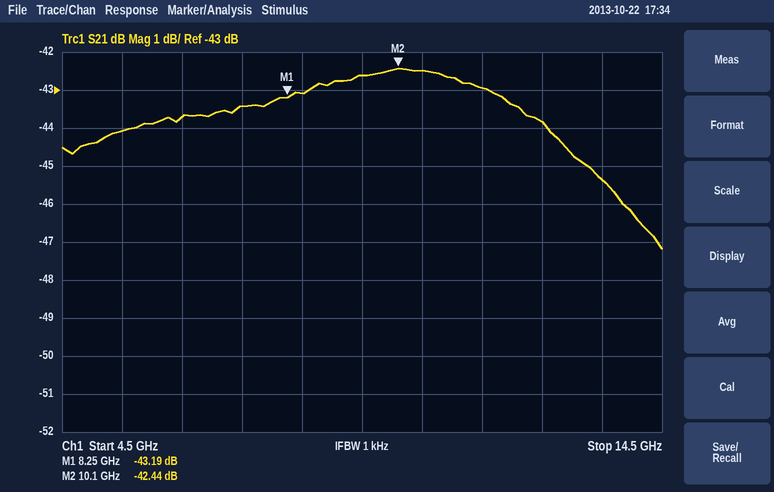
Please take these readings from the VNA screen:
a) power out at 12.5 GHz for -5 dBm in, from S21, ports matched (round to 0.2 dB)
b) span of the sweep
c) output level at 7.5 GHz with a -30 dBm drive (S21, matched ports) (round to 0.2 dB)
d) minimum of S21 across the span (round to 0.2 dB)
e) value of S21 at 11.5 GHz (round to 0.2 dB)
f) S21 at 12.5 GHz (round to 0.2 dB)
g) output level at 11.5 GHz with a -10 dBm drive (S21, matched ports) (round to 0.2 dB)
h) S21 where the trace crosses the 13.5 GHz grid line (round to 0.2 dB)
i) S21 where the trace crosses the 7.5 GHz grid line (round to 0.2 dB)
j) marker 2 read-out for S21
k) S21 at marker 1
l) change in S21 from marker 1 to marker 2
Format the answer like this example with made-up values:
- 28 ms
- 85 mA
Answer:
- -48.8 dBm
- 10 GHz
- -73.4 dBm
- -47.2 dB
- -43.0 dB
- -43.8 dB
- -53.0 dBm
- -45.4 dB
- -43.4 dB
- -42.44 dB
- -43.19 dB
- 0.75 dB
